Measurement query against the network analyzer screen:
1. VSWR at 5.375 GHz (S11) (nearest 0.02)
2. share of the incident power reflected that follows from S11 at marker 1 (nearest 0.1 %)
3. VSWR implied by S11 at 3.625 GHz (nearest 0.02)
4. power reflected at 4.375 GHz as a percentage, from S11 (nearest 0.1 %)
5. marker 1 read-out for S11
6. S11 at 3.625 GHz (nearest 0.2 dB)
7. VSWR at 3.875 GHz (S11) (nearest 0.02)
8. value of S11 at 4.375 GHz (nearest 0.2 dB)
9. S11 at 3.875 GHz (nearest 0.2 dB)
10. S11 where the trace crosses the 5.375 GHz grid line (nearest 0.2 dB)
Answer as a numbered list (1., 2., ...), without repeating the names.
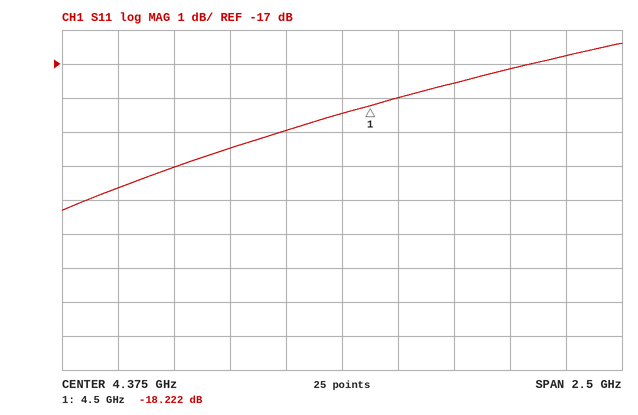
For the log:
1. 1.34
2. 1.5 %
3. 1.22
4. 1.4 %
5. -18.222 dB
6. -20.0 dB
7. 1.24
8. -18.4 dB
9. -19.4 dB
10. -16.8 dB
